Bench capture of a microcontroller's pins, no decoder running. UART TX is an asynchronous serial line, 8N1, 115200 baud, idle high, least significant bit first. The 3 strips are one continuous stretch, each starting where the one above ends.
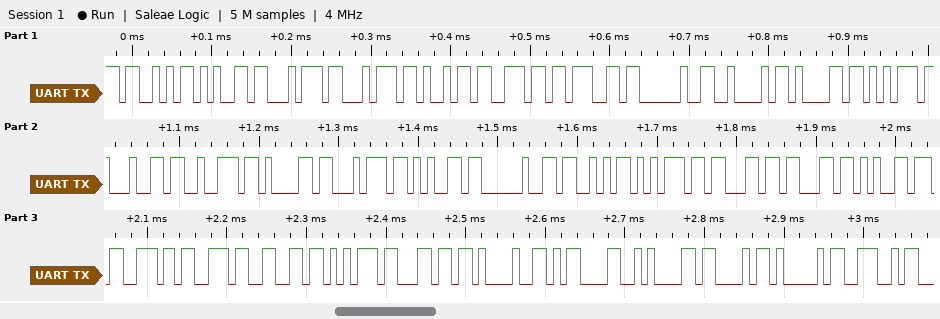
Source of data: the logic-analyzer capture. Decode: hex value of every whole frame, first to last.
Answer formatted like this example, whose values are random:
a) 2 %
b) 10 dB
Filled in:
a) 53 65 74 74 69 6E 67 20 42 61 75 64 72 61 74 65 20 53 75 63 63 65 73 73 66 75 6C 21 0D 0A 43 41 4E
